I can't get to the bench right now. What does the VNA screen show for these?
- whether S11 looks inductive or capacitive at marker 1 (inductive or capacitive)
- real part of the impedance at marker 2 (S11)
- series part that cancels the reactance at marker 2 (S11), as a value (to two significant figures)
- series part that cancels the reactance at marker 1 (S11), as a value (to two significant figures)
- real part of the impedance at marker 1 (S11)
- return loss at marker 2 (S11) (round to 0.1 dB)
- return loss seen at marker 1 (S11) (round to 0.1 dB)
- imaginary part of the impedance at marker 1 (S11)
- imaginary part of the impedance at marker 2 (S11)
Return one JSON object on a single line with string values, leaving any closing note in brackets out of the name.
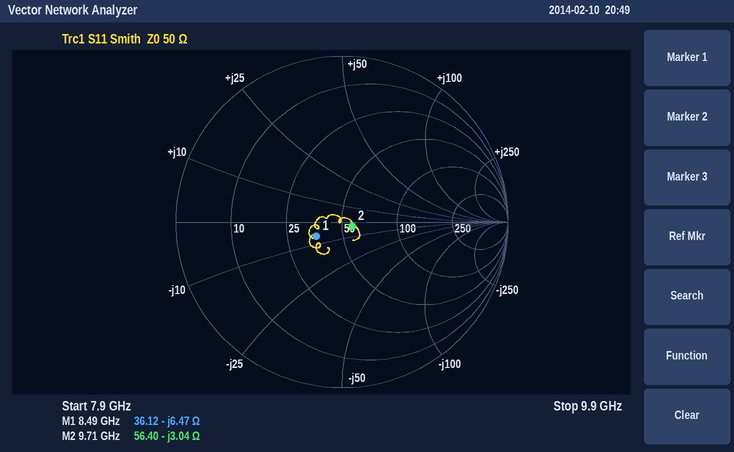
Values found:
{"whether S11 looks inductive or capacitive at marker 1": "capacitive", "real part of the impedance at marker 2": "56.40 Ω", "series part that cancels the reactance at marker 2 (S11), as a value": "50 pH", "series part that cancels the reactance at marker 1 (S11), as a value": "120 pH", "real part of the impedance at marker 1": "36.12 Ω", "return loss at marker 2 (S11)": "23.5 dB", "return loss seen at marker 1 (S11)": "15.0 dB", "imaginary part of the impedance at marker 1": "-6.47 Ω", "imaginary part of the impedance at marker 2": "-3.04 Ω"}
